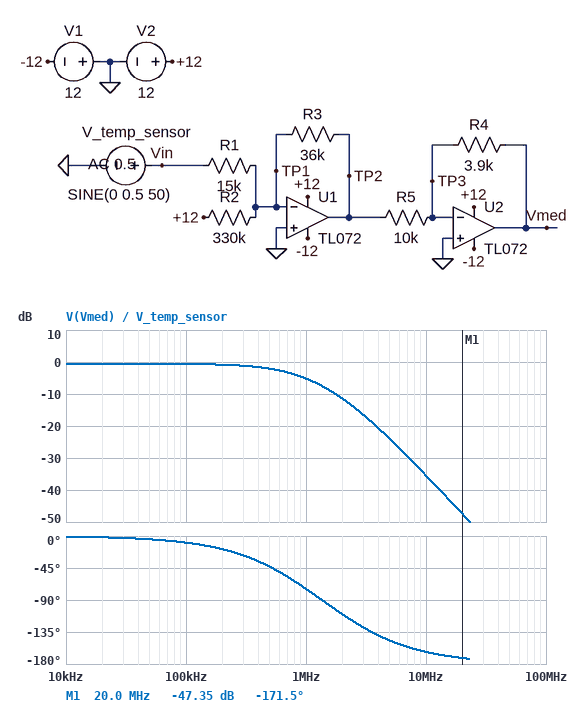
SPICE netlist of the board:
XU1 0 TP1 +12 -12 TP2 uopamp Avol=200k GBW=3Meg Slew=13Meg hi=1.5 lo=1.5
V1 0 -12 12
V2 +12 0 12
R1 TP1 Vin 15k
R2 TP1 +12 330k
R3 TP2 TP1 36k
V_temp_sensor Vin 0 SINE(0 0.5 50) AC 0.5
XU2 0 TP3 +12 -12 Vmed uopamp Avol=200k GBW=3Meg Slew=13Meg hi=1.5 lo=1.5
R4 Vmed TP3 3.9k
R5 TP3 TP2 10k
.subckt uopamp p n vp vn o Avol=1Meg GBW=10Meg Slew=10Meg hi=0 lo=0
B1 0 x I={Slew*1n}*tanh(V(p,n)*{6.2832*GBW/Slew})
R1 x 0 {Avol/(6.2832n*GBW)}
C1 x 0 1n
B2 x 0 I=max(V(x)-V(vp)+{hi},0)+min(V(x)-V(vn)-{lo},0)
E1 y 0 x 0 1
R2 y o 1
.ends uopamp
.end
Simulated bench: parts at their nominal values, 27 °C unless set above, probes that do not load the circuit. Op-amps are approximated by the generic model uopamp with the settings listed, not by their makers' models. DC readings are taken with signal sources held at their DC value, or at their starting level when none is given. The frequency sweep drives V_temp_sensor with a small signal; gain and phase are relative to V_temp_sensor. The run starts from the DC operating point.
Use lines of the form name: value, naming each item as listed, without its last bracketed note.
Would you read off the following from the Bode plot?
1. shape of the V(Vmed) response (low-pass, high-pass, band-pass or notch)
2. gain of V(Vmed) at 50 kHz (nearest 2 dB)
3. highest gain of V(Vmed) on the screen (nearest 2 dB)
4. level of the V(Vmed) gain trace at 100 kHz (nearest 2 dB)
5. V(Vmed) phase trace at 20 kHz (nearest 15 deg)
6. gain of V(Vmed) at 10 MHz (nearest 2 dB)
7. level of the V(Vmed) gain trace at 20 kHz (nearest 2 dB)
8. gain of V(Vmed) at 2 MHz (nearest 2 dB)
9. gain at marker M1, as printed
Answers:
shape of the V(Vmed) response: low-pass
gain of V(Vmed) at 50 kHz: 0 dB
highest gain of V(Vmed) on the screen: 0 dB
level of the V(Vmed) gain trace at 100 kHz: 0 dB
V(Vmed) phase trace at 20 kHz: 0 deg
gain of V(Vmed) at 10 MHz: -36 dB
level of the V(Vmed) gain trace at 20 kHz: 0 dB
gain of V(Vmed) at 2 MHz: -12 dB
gain at marker M1, as printed: -47.35 dB
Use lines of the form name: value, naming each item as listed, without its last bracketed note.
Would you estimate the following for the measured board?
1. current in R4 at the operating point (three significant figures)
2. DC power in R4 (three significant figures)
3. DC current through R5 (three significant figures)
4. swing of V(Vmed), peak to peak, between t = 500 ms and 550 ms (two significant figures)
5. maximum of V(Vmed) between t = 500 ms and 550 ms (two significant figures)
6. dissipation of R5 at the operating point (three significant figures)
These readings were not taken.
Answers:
current in R4 at the operating point: 131 µA
DC power in R4: 66.8 µW
DC current through R5: 131 µA
swing of V(Vmed), peak to peak, between t = 500 ms and 550 ms: 940 mV
maximum of V(Vmed) between t = 500 ms and 550 ms: 980 mV
dissipation of R5 at the operating point: 171 µW
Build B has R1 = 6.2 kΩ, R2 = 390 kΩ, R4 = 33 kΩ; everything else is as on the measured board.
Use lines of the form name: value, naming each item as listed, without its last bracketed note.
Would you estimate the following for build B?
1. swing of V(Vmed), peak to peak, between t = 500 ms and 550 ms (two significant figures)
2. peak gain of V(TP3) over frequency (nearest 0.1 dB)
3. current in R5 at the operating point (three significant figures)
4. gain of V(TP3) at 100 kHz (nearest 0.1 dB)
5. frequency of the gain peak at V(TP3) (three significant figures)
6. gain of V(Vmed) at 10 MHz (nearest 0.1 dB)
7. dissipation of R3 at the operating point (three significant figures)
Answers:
swing of V(Vmed), peak to peak, between t = 500 ms and 550 ms: 16 V
peak gain of V(TP3) over frequency: 4.7 dB
current in R5 at the operating point: 111 µA
gain of V(TP3) at 100 kHz: -4.2 dB
frequency of the gain peak at V(TP3): 551 kHz
gain of V(Vmed) at 10 MHz: -24.7 dB
dissipation of R3 at the operating point: 34.1 µW
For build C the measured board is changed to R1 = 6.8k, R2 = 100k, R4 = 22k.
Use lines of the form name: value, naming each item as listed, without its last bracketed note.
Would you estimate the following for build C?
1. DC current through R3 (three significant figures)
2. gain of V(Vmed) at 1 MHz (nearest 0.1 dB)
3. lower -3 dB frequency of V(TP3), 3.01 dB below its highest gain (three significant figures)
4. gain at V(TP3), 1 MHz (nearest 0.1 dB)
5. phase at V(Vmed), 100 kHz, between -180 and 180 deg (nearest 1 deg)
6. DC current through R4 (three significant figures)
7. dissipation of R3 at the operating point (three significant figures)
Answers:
DC current through R3: 120 µA
gain of V(Vmed) at 1 MHz: 10.3 dB
lower -3 dB frequency of V(TP3), 3.01 dB below its highest gain: 257 kHz
gain at V(TP3), 1 MHz: 0.8 dB
phase at V(Vmed), 100 kHz, between -180 and 180 deg: -19 deg
DC current through R4: 432 µA
dissipation of R3 at the operating point: 518 µW
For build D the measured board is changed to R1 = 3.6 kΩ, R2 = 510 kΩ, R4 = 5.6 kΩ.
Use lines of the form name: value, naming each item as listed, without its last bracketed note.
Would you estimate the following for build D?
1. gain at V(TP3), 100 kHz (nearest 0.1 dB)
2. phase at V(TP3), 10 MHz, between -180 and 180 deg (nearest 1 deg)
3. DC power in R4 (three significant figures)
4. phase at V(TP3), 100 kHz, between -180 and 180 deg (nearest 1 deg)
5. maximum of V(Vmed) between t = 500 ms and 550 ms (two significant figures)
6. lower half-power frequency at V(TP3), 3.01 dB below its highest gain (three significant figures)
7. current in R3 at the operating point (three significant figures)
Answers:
gain at V(TP3), 100 kHz: -15.1 dB
phase at V(TP3), 10 MHz, between -180 and 180 deg: 102 deg
DC power in R4: 40.2 µW
phase at V(TP3), 100 kHz, between -180 and 180 deg: -113 deg
maximum of V(Vmed) between t = 500 ms and 550 ms: 3.3 V
lower half-power frequency at V(TP3), 3.01 dB below its highest gain: 216 kHz
current in R3 at the operating point: 23.5 µA
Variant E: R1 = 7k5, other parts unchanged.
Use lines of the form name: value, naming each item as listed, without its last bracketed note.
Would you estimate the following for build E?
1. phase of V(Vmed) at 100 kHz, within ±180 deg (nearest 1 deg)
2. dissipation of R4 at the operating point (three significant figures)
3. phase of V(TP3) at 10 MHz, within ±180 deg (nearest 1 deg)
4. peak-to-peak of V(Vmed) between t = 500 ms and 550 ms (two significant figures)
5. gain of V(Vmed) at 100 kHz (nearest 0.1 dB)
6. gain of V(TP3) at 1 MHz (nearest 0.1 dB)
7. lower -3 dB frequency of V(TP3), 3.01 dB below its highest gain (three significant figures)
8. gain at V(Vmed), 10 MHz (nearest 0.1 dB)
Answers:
phase of V(Vmed) at 100 kHz, within ±180 deg: -14 deg
dissipation of R4 at the operating point: 66.8 µW
phase of V(TP3) at 10 MHz, within ±180 deg: 105 deg
peak-to-peak of V(Vmed) between t = 500 ms and 550 ms: 1.9 V
gain of V(Vmed) at 100 kHz: 5.3 dB
gain of V(TP3) at 1 MHz: -11.8 dB
lower -3 dB frequency of V(TP3), 3.01 dB below its highest gain: 362 kHz
gain at V(Vmed), 10 MHz: -34.0 dB
